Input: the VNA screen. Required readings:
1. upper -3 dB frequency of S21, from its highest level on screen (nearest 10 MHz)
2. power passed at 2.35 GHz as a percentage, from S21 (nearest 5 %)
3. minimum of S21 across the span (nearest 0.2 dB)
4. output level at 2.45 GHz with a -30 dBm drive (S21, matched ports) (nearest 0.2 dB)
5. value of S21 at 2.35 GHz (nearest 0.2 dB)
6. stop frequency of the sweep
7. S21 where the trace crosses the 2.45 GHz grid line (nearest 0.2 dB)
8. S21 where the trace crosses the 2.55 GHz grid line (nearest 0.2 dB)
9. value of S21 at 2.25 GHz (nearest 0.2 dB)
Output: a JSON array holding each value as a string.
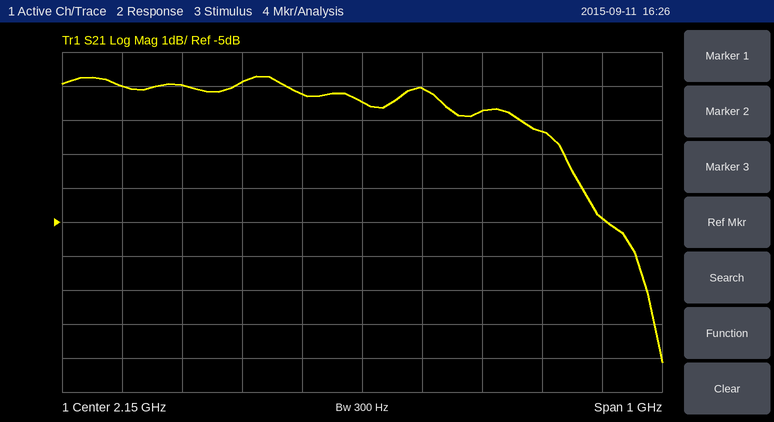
["2.51 GHz", "65 %", "-9.2 dB", "-32.4 dBm", "-1.8 dB", "2.65 GHz", "-2.4 dB", "-4.8 dB", "-1.0 dB"]
